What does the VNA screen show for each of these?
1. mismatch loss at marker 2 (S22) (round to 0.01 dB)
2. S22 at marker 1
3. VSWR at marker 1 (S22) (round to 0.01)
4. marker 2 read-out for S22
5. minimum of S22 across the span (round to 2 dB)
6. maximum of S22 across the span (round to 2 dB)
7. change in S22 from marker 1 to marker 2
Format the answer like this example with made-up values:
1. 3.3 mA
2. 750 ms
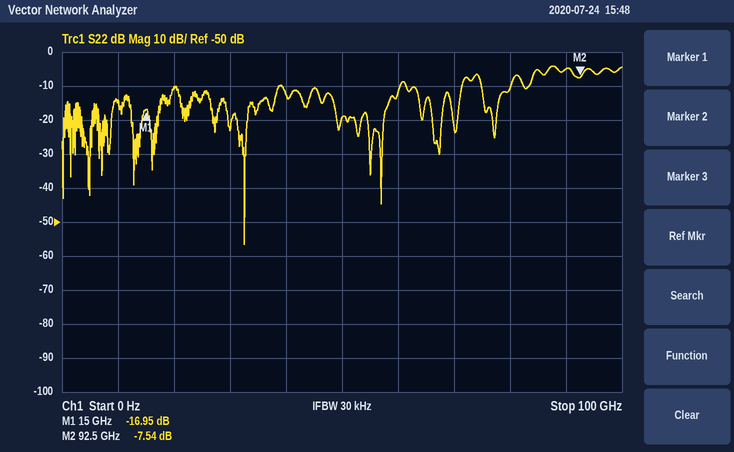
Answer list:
1. 0.84 dB
2. -16.95 dB
3. 1.33
4. -7.54 dB
5. -56 dB
6. -4 dB
7. 9.41 dB
